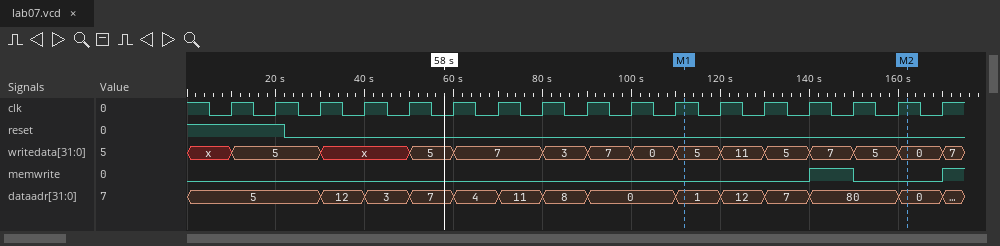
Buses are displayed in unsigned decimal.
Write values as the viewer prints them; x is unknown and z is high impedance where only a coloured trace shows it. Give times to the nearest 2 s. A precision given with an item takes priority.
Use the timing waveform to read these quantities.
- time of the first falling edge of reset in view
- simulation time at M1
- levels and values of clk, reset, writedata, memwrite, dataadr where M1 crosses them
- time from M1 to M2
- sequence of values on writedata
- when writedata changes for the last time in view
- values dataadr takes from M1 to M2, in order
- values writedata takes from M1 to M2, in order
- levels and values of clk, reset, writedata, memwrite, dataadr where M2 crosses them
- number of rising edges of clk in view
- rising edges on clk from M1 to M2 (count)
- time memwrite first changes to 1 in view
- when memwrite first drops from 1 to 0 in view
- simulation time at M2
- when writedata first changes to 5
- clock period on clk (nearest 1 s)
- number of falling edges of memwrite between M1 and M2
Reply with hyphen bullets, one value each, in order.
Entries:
- 22 s
- 112 s
- clk=1, reset=0, writedata=5, memwrite=0, dataadr=1
- 50 s
- x, 5, x, 5, 7, 3, 7, 0, 5, 11, 5, 7, 5, 0, 7
- 170 s
- 1, 12, 7, 80, 0
- 5, 11, 5, 7, 5, 0
- clk=1, reset=0, writedata=0, memwrite=0, dataadr=0
- 17
- 5
- 140 s
- 150 s
- 162 s
- 10 s
- 10 s
- 1
